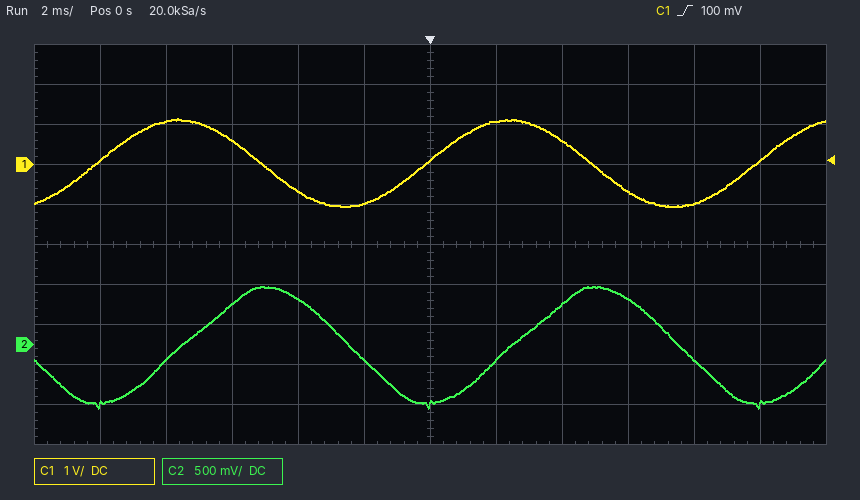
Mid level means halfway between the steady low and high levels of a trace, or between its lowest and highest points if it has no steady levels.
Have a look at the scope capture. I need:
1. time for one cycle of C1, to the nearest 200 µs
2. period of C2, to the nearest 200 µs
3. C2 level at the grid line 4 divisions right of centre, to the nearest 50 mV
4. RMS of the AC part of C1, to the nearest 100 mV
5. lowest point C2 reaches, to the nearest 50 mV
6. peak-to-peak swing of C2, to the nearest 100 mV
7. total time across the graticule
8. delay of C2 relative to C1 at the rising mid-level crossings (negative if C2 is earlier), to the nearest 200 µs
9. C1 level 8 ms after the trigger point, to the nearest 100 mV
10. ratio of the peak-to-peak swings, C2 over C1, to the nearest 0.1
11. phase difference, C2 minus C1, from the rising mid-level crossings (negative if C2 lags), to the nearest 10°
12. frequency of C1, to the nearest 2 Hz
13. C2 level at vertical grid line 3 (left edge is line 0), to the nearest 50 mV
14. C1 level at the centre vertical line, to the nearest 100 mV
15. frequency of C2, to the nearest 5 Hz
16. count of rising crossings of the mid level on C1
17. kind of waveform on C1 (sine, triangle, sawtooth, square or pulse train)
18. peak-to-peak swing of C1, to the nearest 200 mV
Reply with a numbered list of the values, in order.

1. 10.0 ms
2. 10.0 ms
3. -200 mV
4. 800 mV
5. -800 mV
6. 1.50 V
7. 24 ms
8. +2.4 ms
9. -1.0 V
10. 0.7
11. -90°
12. 100 Hz
13. 500 mV
14. 100 mV
15. 100 Hz
16. 3
17. sine
18. 2.2 V
